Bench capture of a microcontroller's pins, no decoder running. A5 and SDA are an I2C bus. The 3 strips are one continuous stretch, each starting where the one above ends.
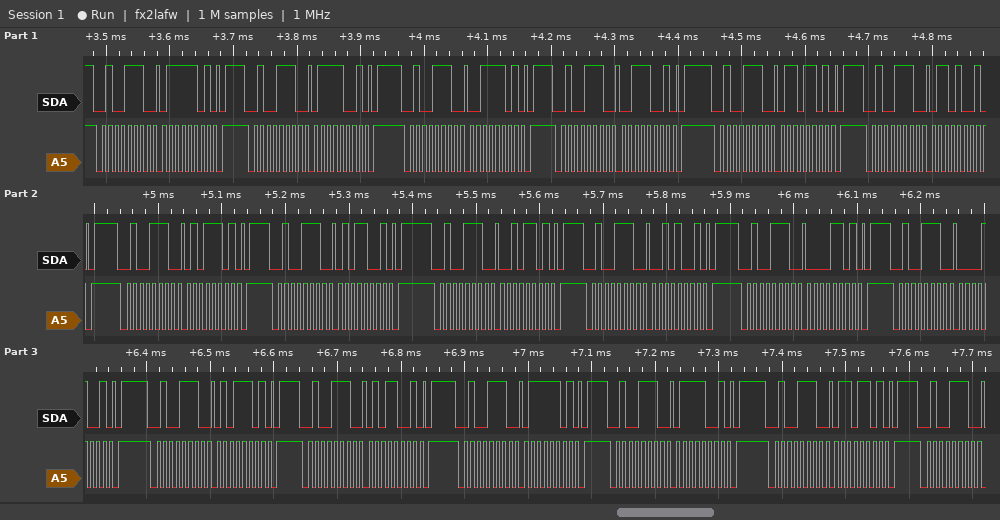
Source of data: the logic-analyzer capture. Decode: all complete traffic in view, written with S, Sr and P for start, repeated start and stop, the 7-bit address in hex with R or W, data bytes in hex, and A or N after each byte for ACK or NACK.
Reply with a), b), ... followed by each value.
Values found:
a) S 27W A 7D A P S 27W A 79 A P S 27W A 3D A P S 27W A 39 A P S 27W A 6D A P S 27W A 69 A P S 27W A 5D A P S 27W A 59 A P S 27W A 2D A P S 27W A 29 A P S 27W A 0D A P S 27W A 09 A P S 27W A 5D A P S 27W A 59 A P S 27W A 7D A P S 27W A 79 A P S 27W A 6D A P S 27W A
